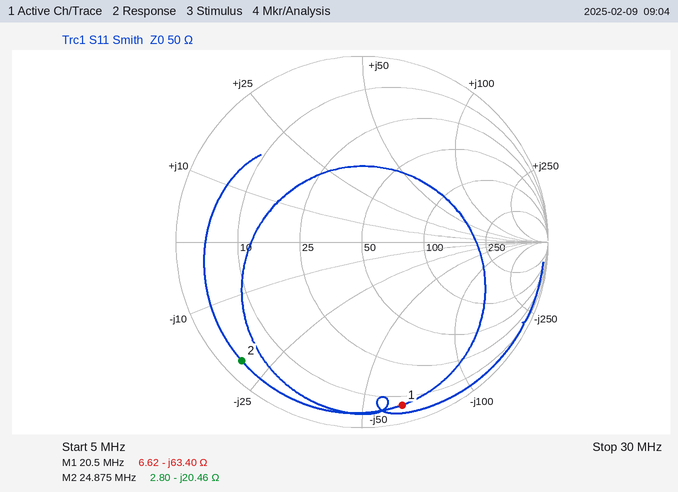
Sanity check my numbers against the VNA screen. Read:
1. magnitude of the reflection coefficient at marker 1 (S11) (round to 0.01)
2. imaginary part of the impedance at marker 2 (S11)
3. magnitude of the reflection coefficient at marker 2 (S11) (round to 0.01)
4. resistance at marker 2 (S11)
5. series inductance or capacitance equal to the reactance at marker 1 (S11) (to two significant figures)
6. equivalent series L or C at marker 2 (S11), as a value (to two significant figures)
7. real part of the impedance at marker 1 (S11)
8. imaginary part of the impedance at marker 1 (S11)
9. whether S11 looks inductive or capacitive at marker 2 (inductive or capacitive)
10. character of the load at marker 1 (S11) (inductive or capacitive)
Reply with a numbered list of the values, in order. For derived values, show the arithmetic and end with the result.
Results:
1. 0.90
2. -20.46 Ω
3. 0.91
4. 2.80 Ω
5. C = 1/(2π × 20.5 MHz × 63.4 Ω) ≈ 122 pF, so 120 pF to two significant figures
6. C = 1/(2π × 24.875 MHz × 20.46 Ω) ≈ 313 pF, so 310 pF to two significant figures
7. 6.62 Ω
8. -63.40 Ω
9. capacitive
10. capacitive
